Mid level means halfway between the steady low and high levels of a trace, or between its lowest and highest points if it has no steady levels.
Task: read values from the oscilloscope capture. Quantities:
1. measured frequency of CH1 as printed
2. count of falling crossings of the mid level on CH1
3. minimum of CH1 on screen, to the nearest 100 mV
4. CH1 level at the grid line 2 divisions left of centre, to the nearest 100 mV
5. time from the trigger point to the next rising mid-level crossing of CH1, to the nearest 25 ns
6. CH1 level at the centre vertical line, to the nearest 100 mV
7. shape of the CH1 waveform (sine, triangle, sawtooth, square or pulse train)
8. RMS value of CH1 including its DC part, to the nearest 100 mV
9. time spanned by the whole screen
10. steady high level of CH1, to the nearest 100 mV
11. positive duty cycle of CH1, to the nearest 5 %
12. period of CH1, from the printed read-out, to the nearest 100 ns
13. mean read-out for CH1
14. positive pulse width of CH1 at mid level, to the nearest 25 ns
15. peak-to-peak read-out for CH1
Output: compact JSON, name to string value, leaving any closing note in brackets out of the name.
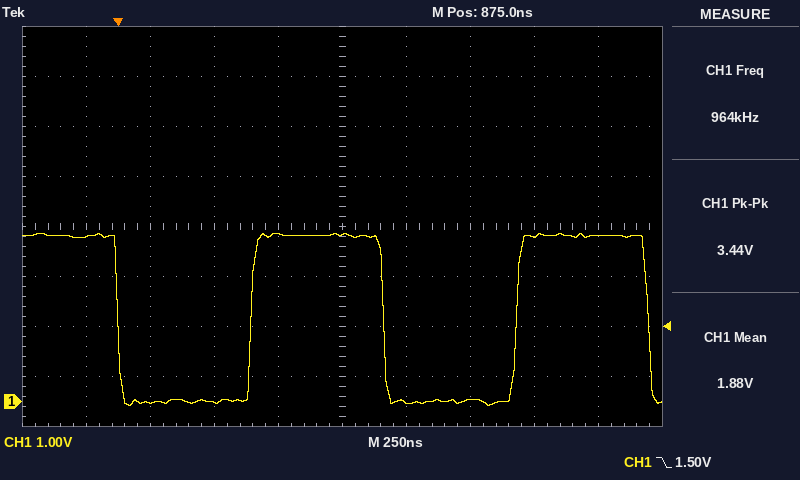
{"measured frequency of CH1 as printed": "964 kHz", "count of falling crossings of the mid level on CH1": "3", "minimum of CH1 on screen, to the nearest 100 mV": "-100 mV", "CH1 level at the grid line 2 divisions left of centre, to the nearest 100 mV": "0.0 V", "time from the trigger point to the next rising mid-level crossing of CH1, to the nearest 25 ns": "525 ns", "CH1 level at the centre vertical line, to the nearest 100 mV": "3.3 V", "shape of the CH1 waveform": "square", "RMS value of CH1 including its DC part, to the nearest 100 mV": "2.3 V", "time spanned by the whole screen": "2.5 µs", "steady high level of CH1, to the nearest 100 mV": "3.3 V", "positive duty cycle of CH1, to the nearest 5 %": "50 %", "period of CH1, from the printed read-out, to the nearest 100 ns": "1.0 µs", "mean read-out for CH1": "1.88 V", "positive pulse width of CH1 at mid level, to the nearest 25 ns": "525 ns", "peak-to-peak read-out for CH1": "3.44 V"}
